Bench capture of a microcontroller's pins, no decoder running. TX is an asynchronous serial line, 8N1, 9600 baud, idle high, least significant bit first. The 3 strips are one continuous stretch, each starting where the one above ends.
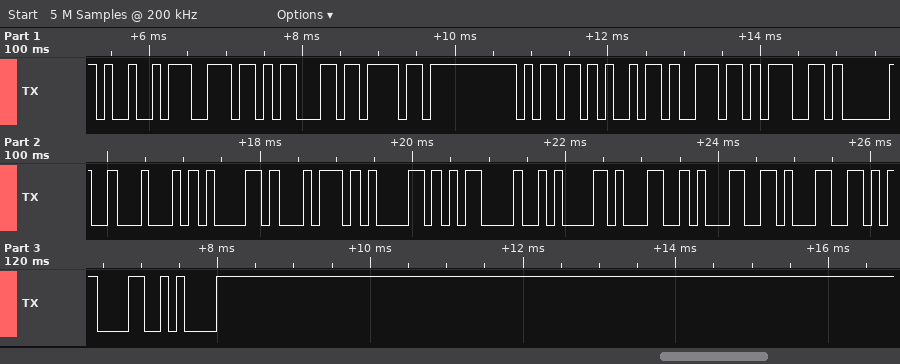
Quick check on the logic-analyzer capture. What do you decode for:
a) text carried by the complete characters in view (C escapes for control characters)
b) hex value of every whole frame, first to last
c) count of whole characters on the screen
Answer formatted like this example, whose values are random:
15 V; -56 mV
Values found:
"Incoming Data\r\n111\r\n"; 0x49 0x6E 0x63 0x6F 0x6D 0x69 0x6E 0x67 0x20 0x44 0x61 0x74 0x61 0x0D 0x0A 0x31 0x31 0x31 0x0D 0x0A; 20
